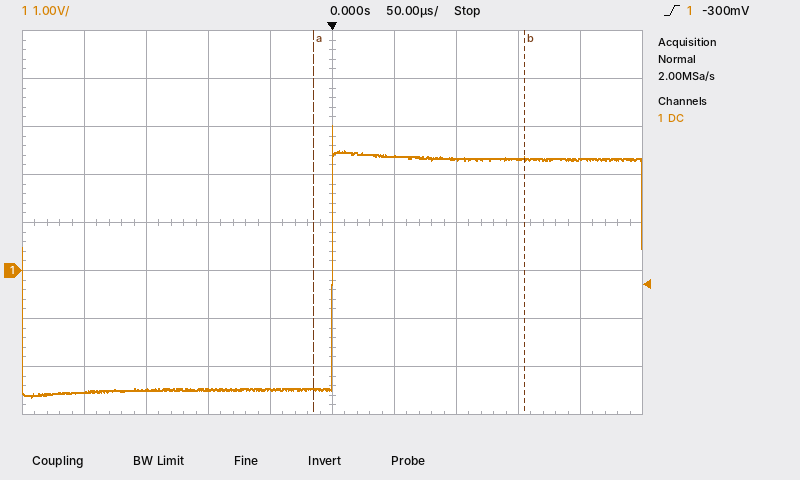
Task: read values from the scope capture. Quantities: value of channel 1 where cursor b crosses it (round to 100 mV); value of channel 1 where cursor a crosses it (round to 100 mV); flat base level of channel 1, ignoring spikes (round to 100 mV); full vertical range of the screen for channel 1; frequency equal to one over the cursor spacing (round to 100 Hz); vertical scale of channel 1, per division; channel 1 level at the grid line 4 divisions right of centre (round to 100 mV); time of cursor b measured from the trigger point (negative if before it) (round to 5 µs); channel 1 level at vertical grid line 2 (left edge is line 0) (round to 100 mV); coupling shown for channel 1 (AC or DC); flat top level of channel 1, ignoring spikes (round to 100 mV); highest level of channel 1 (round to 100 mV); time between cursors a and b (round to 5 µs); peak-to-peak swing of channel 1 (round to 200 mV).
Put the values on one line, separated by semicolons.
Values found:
2.3 V; -2.5 V; -2.5 V; 8 V; 5.9 kHz; 1 V; 2.3 V; +155 µs; -2.5 V; DC; 2.3 V; 3.0 V; 170 µs; 5.6 V
